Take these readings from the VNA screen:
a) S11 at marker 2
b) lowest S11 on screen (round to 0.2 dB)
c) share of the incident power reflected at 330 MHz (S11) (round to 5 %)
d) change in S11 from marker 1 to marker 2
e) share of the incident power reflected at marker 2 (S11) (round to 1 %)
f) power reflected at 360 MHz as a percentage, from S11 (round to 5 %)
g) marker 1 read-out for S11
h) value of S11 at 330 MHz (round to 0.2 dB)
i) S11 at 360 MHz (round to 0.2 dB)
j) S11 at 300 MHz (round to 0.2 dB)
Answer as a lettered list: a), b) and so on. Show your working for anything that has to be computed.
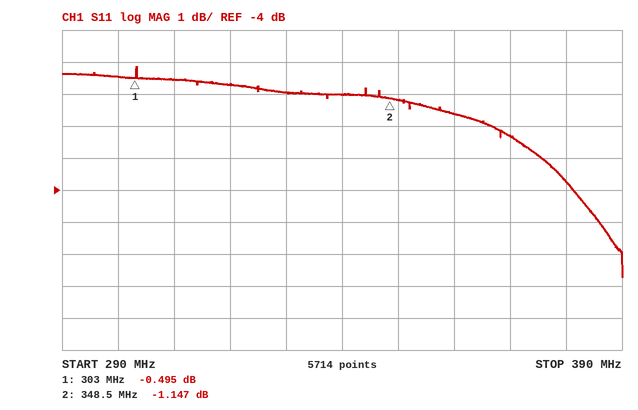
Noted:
a) -1.147 dB
b) -6.8 dB
c) 10^(-1/10) ≈ 79.4 %, so 80 % to the nearest 5 %
d) -1.147 − (-0.495) = -0.652 dB
e) 10^(-1.147/10) ≈ 77 %
f) 10^(-1.6/10) ≈ 69.2 %, so 70 % to the nearest 5 %
g) -0.495 dB
h) -1.0 dB
i) -1.6 dB
j) -0.4 dB
